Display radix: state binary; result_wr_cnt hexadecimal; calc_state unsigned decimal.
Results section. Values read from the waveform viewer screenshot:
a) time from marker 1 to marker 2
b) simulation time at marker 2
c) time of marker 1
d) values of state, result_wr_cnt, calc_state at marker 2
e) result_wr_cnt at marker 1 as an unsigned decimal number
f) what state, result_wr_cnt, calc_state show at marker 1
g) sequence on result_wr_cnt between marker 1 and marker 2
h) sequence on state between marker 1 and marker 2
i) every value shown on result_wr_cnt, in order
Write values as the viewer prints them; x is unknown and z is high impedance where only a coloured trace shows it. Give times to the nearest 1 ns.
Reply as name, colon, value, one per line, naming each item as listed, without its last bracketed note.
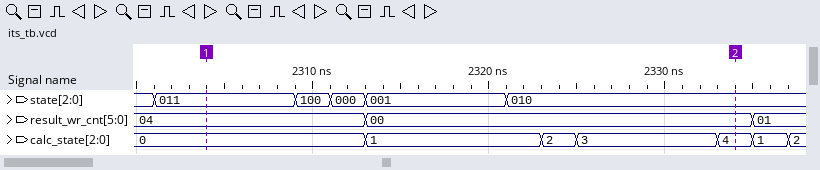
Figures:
time from marker 1 to marker 2: 30 ns
simulation time at marker 2: 2334 ns
time of marker 1: 2304 ns
values of state, result_wr_cnt, calc_state at marker 2: state=010, result_wr_cnt=00, calc_state=4
result_wr_cnt at marker 1 as an unsigned decimal number: 4
what state, result_wr_cnt, calc_state show at marker 1: state=011, result_wr_cnt=04, calc_state=0
sequence on result_wr_cnt between marker 1 and marker 2: 04, 00
sequence on state between marker 1 and marker 2: 011, 100, 000, 001, 010
every value shown on result_wr_cnt, in order: 04, 00, 01
